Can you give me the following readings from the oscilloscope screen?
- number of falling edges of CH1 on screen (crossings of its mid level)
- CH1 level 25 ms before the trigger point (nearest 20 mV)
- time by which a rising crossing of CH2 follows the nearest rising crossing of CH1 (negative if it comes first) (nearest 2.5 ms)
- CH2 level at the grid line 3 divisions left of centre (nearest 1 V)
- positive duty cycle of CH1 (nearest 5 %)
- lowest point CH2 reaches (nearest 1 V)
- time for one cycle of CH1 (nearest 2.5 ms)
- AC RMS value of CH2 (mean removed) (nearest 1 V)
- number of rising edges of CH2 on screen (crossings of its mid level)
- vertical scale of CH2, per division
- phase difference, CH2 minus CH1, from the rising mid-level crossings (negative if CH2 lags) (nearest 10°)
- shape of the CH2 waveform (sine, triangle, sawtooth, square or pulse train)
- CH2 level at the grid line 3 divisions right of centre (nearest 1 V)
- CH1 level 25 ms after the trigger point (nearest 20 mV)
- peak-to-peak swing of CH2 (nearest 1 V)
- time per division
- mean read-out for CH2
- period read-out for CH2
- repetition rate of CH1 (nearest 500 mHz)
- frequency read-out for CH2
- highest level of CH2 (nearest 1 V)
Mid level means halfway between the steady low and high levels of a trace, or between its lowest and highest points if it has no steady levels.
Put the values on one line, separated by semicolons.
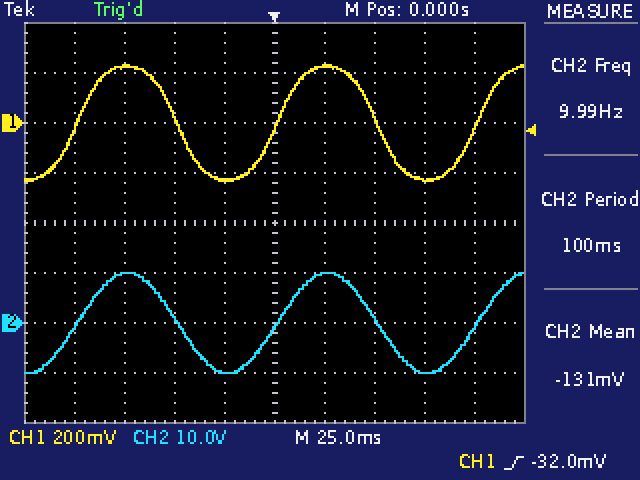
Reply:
2; -220 mV; 0.0 ms; 10 V; 50 %; -10 V; 100.0 ms; 7 V; 3; 10 V; 0°; sine; -10 V; 220 mV; 20 V; 25 ms; -131 mV; 100 ms; 10.0 Hz; 9.99 Hz; 10 V
